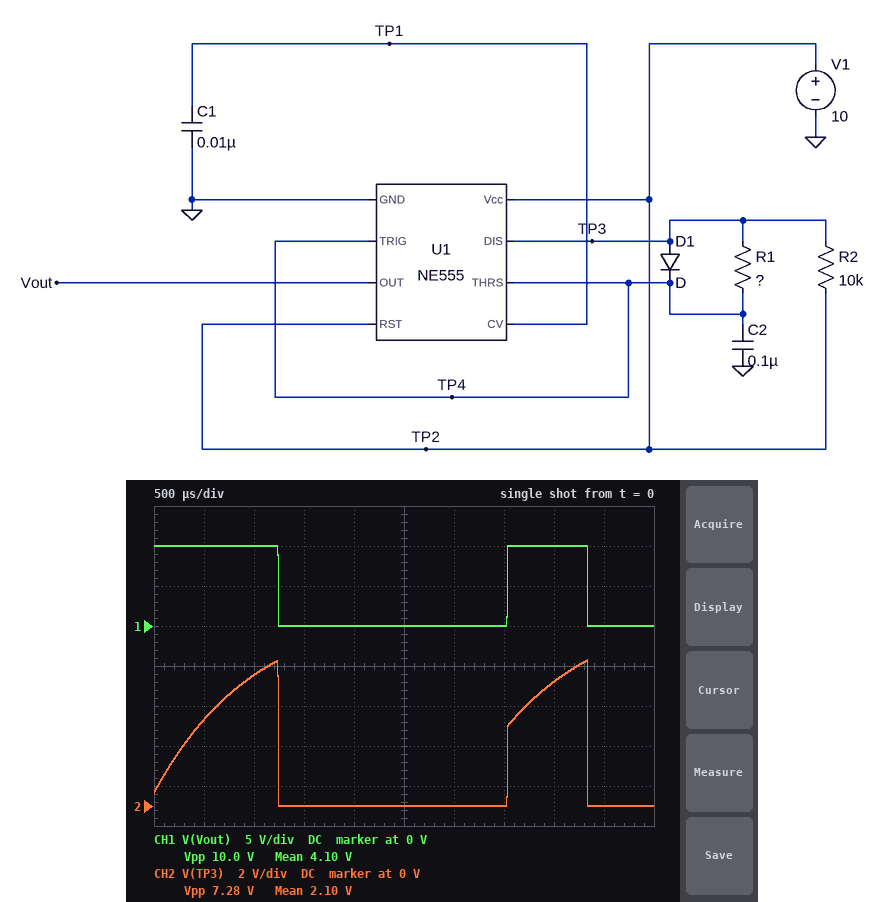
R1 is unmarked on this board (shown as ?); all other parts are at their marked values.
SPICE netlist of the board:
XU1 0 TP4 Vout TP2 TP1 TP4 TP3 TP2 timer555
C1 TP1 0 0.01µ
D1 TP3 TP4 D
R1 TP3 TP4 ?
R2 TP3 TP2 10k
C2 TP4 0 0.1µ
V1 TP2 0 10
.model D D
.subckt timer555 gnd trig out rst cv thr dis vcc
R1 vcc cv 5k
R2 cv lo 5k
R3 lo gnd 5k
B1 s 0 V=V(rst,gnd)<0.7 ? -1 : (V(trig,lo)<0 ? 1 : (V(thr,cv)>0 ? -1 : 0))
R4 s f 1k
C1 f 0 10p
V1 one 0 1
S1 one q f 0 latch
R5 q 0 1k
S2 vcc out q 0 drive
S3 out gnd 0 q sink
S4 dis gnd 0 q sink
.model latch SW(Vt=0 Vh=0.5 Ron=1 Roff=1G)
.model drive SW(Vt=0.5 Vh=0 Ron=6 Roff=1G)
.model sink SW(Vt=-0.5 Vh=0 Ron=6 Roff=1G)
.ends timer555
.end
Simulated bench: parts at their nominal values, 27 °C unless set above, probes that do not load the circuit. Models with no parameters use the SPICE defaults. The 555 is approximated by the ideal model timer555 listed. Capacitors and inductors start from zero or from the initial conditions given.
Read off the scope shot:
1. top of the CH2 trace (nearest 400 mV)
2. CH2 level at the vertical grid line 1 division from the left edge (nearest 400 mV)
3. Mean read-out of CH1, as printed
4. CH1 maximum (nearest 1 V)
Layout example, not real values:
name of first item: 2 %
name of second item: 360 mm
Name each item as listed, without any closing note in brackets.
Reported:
top of the CH2 trace: 7.2 V
CH2 level at the vertical grid line 1 division from the left edge: 4.4 V
Mean read-out of CH1, as printed: 4.10 V
CH1 maximum: 10 V
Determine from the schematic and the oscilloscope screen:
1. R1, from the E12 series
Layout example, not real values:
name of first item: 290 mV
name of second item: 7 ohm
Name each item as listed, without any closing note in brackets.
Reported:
R1, from the E12 series: 33 kΩ
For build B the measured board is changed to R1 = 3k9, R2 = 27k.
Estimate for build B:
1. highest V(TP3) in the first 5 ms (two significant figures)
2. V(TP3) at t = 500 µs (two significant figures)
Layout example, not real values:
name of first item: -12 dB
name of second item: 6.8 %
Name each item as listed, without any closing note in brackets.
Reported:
highest V(TP3) in the first 5 ms: 7.1 V
V(TP3) at t = 500 µs: 2.2 V
